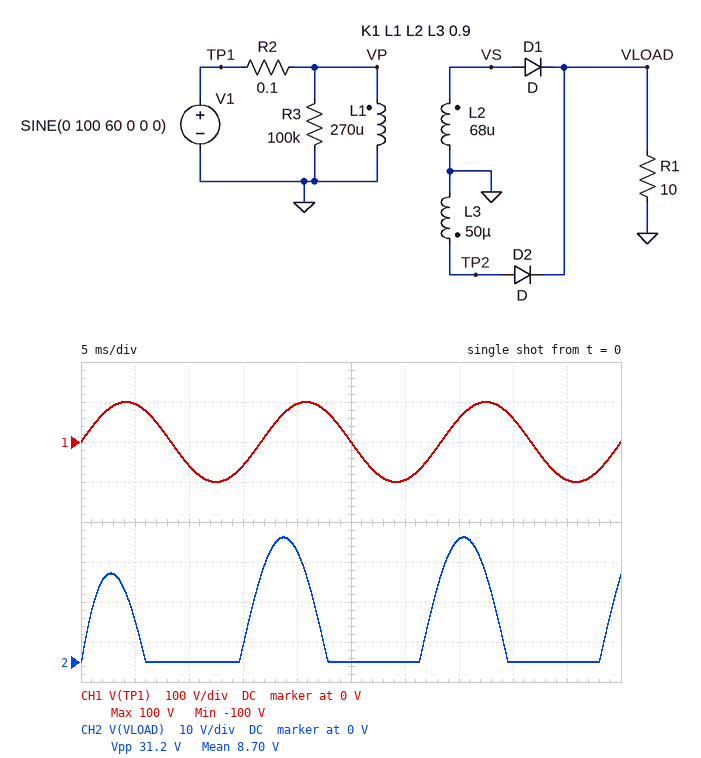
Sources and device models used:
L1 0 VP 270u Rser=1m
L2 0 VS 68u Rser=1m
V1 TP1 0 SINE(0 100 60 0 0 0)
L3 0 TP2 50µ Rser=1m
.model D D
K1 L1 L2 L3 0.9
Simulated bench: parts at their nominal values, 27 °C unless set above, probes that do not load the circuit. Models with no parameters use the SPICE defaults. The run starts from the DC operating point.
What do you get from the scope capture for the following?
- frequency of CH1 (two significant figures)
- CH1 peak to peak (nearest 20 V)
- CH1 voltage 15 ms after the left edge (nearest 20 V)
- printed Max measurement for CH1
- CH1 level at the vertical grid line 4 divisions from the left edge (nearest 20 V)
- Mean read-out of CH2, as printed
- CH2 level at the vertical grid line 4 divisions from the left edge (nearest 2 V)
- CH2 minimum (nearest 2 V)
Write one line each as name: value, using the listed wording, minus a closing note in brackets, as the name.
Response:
frequency of CH1: 60 Hz
CH1 peak to peak: 200 V
CH1 voltage 15 ms after the left edge: -60 V
printed Max measurement for CH1: 100 V
CH1 level at the vertical grid line 4 divisions from the left edge: 100 V
Mean read-out of CH2, as printed: 8.70 V
CH2 level at the vertical grid line 4 divisions from the left edge: 28 V
CH2 minimum: 0 V
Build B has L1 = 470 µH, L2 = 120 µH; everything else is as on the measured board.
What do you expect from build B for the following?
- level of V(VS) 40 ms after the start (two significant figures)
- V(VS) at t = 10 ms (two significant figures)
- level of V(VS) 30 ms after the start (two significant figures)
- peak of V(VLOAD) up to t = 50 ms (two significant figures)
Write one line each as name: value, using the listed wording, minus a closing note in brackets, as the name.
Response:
level of V(VS) 40 ms after the start: 4.4 V
V(VS) at t = 10 ms: -38 V
level of V(VS) 30 ms after the start: -27 V
peak of V(VLOAD) up to t = 50 ms: 39 V
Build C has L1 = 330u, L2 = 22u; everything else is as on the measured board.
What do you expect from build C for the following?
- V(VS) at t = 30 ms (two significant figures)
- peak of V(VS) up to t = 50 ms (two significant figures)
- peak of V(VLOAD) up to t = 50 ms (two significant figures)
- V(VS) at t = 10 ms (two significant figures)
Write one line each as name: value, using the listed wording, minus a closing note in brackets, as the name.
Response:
V(VS) at t = 30 ms: -9.8 V
peak of V(VS) up to t = 50 ms: 18 V
peak of V(VLOAD) up to t = 50 ms: 26 V
V(VS) at t = 10 ms: -18 V
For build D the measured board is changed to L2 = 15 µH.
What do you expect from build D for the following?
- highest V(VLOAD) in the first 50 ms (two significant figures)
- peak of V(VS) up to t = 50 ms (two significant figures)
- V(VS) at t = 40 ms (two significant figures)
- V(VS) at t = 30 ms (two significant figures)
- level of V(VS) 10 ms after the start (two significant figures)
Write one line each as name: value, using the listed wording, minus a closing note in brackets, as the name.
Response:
highest V(VLOAD) in the first 50 ms: 27 V
peak of V(VS) up to t = 50 ms: 15 V
V(VS) at t = 40 ms: -2.3 V
V(VS) at t = 30 ms: -6.9 V
level of V(VS) 10 ms after the start: -15 V
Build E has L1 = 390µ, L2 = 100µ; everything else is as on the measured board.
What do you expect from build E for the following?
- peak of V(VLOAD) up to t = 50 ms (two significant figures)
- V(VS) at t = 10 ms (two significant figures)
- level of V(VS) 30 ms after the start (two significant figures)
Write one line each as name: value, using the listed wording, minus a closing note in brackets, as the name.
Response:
peak of V(VLOAD) up to t = 50 ms: 37 V
V(VS) at t = 10 ms: -37 V
level of V(VS) 30 ms after the start: -23 V
